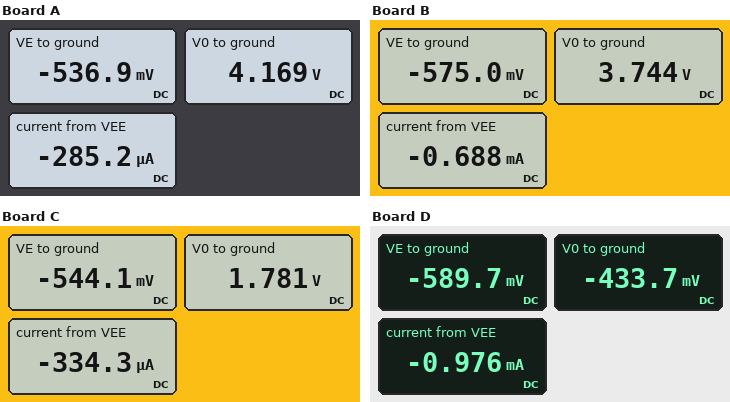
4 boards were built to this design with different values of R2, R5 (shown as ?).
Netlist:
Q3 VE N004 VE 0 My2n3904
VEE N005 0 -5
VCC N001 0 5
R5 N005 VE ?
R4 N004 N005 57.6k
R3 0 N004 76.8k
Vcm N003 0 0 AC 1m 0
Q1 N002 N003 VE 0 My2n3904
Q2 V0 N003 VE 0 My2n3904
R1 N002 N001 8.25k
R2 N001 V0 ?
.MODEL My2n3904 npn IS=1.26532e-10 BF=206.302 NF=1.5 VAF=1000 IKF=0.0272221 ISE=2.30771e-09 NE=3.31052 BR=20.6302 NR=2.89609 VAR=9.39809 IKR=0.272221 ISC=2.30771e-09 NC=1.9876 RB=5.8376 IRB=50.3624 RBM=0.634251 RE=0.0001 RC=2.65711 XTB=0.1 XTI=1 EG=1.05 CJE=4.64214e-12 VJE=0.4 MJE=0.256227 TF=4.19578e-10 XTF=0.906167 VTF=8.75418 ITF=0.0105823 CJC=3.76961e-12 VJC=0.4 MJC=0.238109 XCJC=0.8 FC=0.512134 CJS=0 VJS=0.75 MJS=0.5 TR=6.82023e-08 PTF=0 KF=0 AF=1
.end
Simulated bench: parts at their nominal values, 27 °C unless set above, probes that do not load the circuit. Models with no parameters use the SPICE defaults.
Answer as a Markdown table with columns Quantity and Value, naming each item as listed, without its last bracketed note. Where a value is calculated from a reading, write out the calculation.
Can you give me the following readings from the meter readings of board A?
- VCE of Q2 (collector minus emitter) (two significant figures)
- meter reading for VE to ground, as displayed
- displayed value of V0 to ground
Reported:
| Quantity | Value |
|---|---|
| VCE of Q2 (collector minus emitter) | 4.169 V - (-536.9 mV) = 4.7 V |
| meter reading for VE to ground, as displayed | -536.9 mV |
| displayed value of V0 to ground | 4.169 V |
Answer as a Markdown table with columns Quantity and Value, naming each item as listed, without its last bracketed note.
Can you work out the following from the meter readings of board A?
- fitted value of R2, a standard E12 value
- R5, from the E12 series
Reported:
| Quantity | Value |
|---|---|
| fitted value of R2, a standard E12 value | 6.8 kΩ |
| R5, from the E12 series | 18 kΩ |
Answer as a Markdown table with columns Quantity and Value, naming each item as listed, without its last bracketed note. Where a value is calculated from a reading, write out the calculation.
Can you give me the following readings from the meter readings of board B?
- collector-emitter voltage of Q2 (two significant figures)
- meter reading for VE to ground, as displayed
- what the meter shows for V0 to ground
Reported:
| Quantity | Value |
|---|---|
| collector-emitter voltage of Q2 | 3.744 V - (-575 mV) = 4.3 V |
| meter reading for VE to ground, as displayed | -575.0 mV |
| what the meter shows for V0 to ground | 3.744 V |
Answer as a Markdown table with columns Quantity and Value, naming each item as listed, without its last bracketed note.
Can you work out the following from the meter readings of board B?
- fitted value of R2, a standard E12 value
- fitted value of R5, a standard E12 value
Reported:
| Quantity | Value |
|---|---|
| fitted value of R2, a standard E12 value | 3.9 kΩ |
| fitted value of R5, a standard E12 value | 6.8 kΩ |
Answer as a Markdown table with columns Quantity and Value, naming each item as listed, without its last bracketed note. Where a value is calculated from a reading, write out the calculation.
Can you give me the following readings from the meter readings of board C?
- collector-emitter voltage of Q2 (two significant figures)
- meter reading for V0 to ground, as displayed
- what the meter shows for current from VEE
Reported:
| Quantity | Value |
|---|---|
| collector-emitter voltage of Q2 | 1.781 V - (-544.1 mV) = 2.3 V |
| meter reading for V0 to ground, as displayed | 1.781 V |
| what the meter shows for current from VEE | -334.3 µA |
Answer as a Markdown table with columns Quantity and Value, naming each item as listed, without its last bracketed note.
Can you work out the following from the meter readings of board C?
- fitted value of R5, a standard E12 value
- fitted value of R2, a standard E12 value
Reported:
| Quantity | Value |
|---|---|
| fitted value of R5, a standard E12 value | 15 kΩ |
| fitted value of R2, a standard E12 value | 22 kΩ |
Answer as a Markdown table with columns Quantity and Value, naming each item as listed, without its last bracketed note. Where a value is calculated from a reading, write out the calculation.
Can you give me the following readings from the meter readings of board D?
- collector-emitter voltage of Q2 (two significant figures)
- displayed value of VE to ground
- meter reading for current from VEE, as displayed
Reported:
| Quantity | Value |
|---|---|
| collector-emitter voltage of Q2 | -433.7 mV - (-589.7 mV) = 160 mV |
| displayed value of VE to ground | -589.7 mV |
| meter reading for current from VEE, as displayed | -0.976 mA |
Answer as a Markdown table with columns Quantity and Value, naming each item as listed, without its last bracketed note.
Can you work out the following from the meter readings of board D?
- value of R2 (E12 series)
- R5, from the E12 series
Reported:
| Quantity | Value |
|---|---|
| value of R2 | 12 kΩ |
| R5, from the E12 series | 4.7 kΩ |
